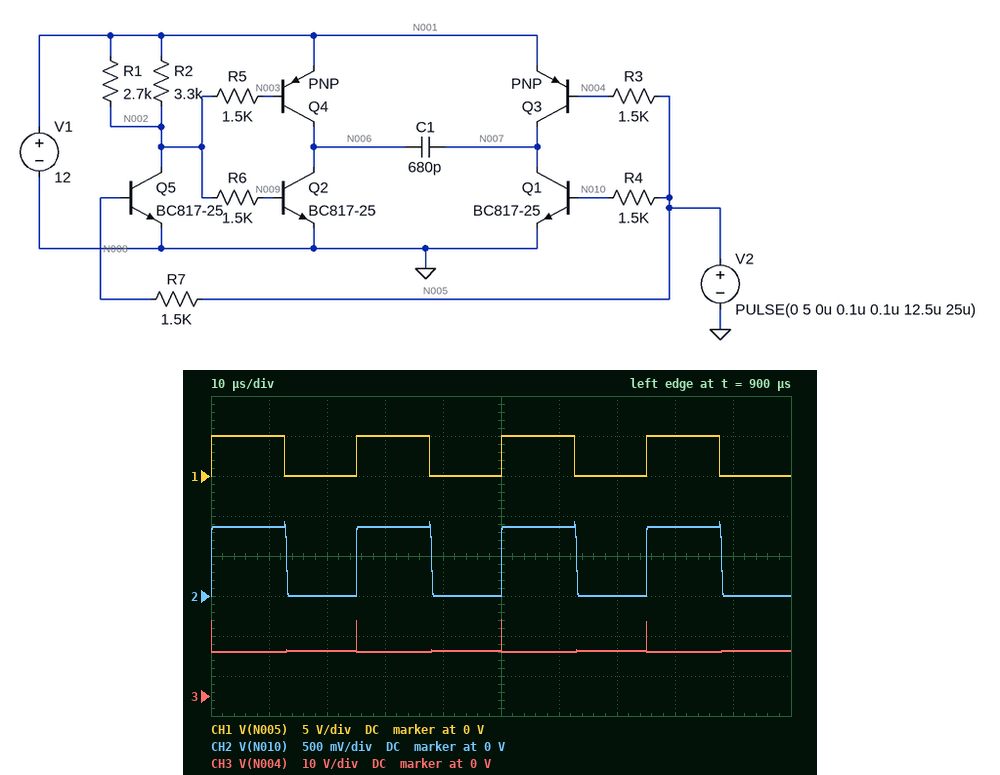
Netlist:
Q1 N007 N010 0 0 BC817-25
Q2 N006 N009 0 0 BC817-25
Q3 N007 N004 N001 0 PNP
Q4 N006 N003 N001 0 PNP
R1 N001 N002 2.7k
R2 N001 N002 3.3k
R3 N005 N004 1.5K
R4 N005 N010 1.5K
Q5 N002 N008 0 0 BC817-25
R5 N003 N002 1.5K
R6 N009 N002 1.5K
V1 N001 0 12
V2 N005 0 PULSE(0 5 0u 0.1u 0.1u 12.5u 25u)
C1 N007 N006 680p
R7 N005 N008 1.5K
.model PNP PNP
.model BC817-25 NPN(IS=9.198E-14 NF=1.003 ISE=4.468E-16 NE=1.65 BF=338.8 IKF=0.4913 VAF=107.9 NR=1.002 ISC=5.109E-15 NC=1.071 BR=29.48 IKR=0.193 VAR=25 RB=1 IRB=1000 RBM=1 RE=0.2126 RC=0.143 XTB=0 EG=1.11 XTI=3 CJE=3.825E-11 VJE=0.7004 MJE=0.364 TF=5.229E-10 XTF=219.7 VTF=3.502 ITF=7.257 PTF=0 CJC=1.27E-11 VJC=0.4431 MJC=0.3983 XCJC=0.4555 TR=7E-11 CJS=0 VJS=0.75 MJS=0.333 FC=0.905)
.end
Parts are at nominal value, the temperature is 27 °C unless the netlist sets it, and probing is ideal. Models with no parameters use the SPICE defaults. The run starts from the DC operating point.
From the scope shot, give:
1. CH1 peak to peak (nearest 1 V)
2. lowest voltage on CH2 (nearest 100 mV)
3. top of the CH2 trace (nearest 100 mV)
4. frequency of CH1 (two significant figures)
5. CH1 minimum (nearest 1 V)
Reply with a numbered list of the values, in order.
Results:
1. 5 V
2. 0 V
3. 900 mV
4. 40 kHz
5. 0 V
